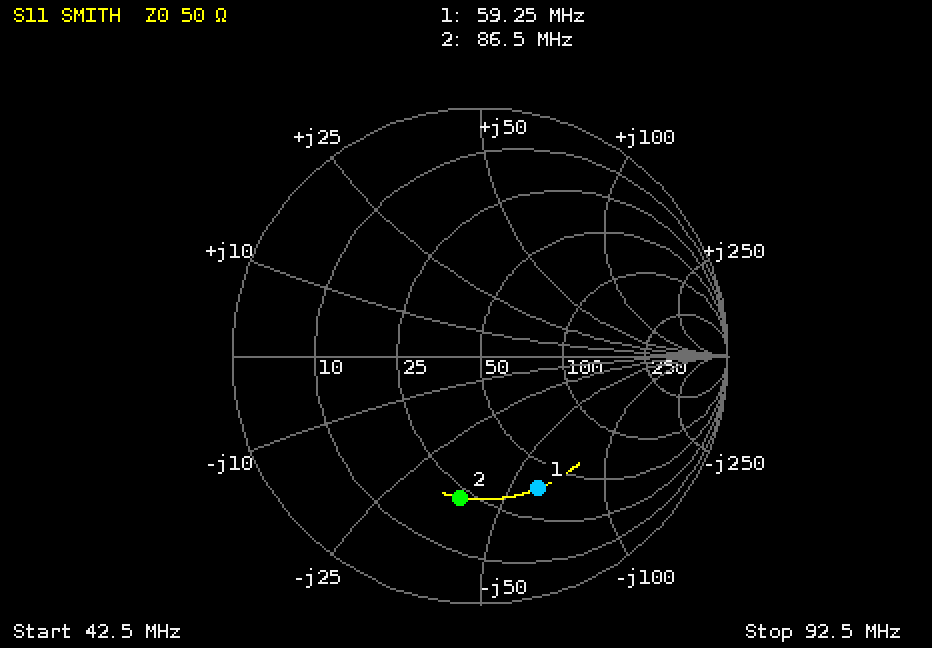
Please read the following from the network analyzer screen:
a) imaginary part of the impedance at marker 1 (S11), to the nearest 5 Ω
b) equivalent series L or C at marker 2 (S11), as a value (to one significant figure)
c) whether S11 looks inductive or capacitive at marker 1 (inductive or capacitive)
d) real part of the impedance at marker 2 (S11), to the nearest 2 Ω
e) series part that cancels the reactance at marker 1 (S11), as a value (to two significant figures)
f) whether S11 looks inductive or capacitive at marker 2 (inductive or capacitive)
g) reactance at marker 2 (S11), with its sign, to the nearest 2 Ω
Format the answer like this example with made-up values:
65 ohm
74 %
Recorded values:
-60 Ω
50 pF
capacitive
22 Ω
160 nH
capacitive
-38 Ω
